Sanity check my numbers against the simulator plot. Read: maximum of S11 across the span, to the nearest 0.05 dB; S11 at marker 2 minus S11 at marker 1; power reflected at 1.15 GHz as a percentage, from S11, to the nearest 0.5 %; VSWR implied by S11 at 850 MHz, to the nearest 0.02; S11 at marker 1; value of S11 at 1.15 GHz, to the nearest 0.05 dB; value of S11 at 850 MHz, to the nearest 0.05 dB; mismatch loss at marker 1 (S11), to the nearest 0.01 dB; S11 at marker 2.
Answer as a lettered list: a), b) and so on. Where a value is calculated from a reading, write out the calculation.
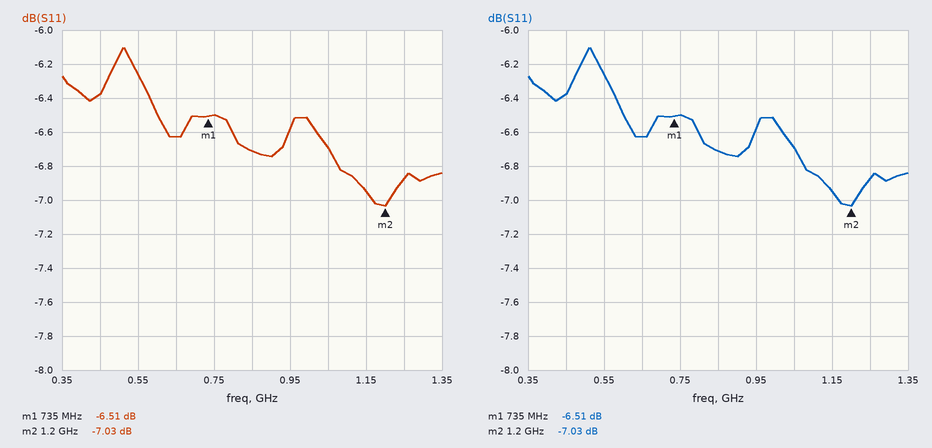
a) -6.10 dB
b) -7.03 − (-6.51) = -0.52 dB
c) 10^(-6.95/10) ≈ 20.2 %, so 20.0 % to the nearest 0.5 %
d) |Γ| = 10^(-6.7/20) = 0.4624; VSWR = (1 + 0.4624)/(1 − 0.4624) ≈ 2.72
e) -6.51 dB
f) -6.95 dB
g) -6.70 dB
h) −10 log10(1 − 10^(-6.51/10)) ≈ 1.10 dB
i) -7.03 dB
